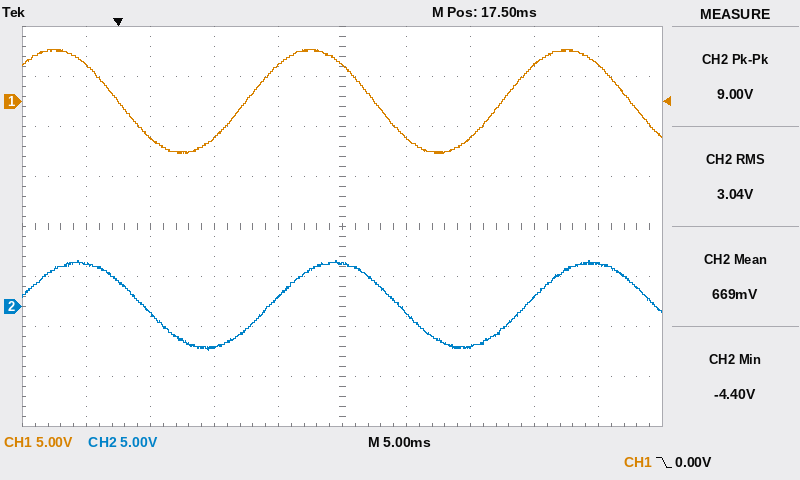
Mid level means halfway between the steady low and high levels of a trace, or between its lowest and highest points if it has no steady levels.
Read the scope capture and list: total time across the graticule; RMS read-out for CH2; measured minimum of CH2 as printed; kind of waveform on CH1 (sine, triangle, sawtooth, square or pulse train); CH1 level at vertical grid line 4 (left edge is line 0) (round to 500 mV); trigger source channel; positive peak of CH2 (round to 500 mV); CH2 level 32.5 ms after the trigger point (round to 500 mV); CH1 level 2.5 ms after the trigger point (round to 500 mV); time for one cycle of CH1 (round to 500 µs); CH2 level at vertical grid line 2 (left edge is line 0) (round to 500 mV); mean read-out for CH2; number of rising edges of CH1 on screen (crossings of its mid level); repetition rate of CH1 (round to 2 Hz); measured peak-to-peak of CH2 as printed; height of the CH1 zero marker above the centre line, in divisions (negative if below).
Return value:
50 ms
3.04 V
-4.40 V
sine
3.5 V
CH1
4.5 V
1.0 V
-3.5 V
20.0 ms
-500 mV
669 mV
2
50 Hz
9.00 V
+2.5 div
